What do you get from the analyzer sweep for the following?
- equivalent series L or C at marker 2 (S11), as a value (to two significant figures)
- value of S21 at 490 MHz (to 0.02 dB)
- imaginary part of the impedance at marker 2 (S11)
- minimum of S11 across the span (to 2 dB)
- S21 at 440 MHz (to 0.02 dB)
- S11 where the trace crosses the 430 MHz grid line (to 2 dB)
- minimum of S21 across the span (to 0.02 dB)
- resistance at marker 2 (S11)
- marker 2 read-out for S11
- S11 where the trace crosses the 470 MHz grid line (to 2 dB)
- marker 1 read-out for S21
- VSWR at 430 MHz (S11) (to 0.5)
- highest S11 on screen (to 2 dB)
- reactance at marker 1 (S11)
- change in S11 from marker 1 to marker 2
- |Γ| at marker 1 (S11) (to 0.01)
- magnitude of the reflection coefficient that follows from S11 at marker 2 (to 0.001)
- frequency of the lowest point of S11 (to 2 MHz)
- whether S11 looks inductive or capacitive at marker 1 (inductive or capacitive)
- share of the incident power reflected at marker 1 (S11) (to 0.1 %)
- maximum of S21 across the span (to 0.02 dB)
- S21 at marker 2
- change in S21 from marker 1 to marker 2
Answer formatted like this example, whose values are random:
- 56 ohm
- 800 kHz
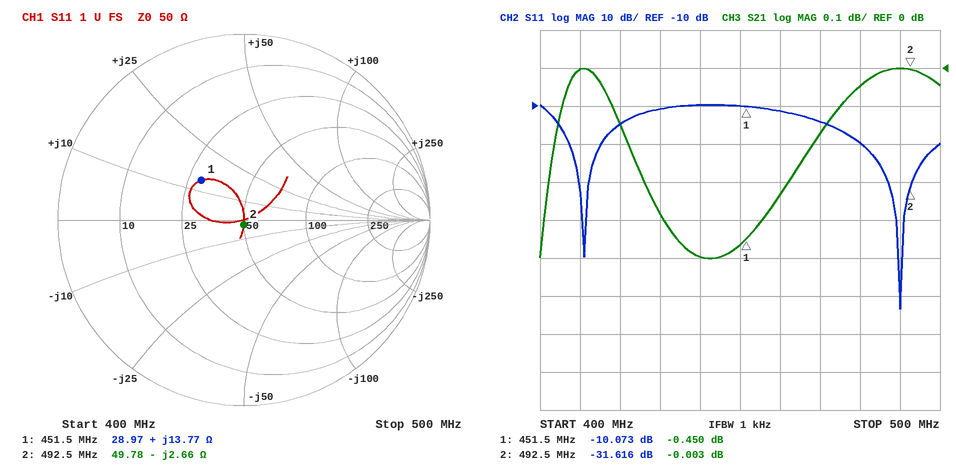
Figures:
- 120 pF
- 0.00 dB
- -2.66 Ω
- -64 dB
- -0.50 dB
- -10 dB
- -0.50 dB
- 49.78 Ω
- -31.616 dB
- -14 dB
- -0.450 dB
- 2.0
- -10 dB
- +13.77 Ω
- -21.543 dB
- 0.31
- 0.026
- 490 MHz
- inductive
- 9.8 %
- 0.00 dB
- -0.003 dB
- 0.447 dB
